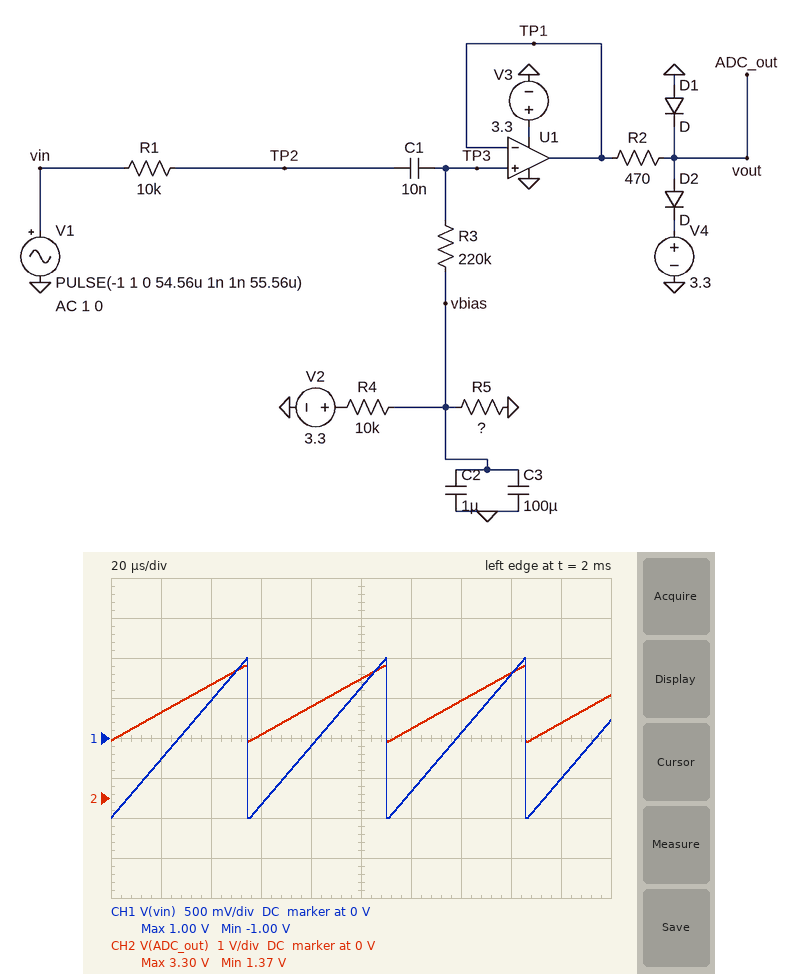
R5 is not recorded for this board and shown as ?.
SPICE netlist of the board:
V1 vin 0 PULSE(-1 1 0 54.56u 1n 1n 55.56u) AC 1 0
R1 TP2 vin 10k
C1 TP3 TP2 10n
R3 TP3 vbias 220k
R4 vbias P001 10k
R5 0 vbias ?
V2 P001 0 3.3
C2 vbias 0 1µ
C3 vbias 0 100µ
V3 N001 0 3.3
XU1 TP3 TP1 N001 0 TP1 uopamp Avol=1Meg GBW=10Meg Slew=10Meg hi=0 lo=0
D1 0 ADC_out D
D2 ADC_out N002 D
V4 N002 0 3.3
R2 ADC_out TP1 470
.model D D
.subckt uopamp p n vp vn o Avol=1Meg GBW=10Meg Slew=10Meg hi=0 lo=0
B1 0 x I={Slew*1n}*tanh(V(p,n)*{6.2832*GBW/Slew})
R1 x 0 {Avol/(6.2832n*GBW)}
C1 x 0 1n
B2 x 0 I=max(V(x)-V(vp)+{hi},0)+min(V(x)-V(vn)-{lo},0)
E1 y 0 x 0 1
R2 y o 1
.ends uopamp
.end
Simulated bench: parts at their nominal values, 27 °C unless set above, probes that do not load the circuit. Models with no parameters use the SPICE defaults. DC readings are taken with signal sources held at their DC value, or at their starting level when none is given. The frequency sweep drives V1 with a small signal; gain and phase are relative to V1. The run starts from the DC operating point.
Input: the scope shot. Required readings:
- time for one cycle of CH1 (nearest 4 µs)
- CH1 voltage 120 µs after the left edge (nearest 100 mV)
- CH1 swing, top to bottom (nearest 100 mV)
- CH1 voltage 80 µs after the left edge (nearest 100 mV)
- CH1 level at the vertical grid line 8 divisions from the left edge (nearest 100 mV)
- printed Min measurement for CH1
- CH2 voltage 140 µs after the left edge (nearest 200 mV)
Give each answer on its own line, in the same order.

56 µs
-700 mV
2.0 V
-100 mV
800 mV
-1.00 V
2.4 V
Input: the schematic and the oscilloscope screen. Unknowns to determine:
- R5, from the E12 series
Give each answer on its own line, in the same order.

15 kΩ
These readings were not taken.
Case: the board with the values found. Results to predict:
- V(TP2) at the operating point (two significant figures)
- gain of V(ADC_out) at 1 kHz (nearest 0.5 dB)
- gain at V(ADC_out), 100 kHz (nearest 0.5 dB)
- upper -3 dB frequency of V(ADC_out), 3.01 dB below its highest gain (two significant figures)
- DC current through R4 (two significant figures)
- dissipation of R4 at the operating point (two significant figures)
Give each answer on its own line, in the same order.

-1.0 V
-0.5 dB
-0.5 dB
10 MHz
130 µA
170 µW
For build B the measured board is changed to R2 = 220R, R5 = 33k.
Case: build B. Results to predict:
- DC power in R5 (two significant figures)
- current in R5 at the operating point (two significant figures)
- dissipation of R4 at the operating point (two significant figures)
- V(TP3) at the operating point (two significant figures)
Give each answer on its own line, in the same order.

190 µW
77 µA
59 µW
2.5 V
